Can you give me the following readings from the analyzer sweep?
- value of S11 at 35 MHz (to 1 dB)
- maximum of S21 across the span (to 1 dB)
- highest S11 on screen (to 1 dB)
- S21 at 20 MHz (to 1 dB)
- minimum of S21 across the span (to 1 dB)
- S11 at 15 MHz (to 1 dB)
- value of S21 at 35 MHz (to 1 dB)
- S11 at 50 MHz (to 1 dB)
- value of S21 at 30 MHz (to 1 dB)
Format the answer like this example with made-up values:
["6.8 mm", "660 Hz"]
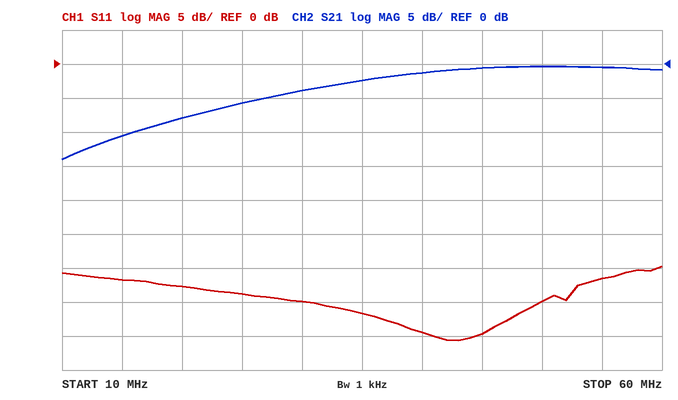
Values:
["-37 dB", "0 dB", "-30 dB", "-8 dB", "-14 dB", "-32 dB", "-2 dB", "-35 dB", "-4 dB"]
